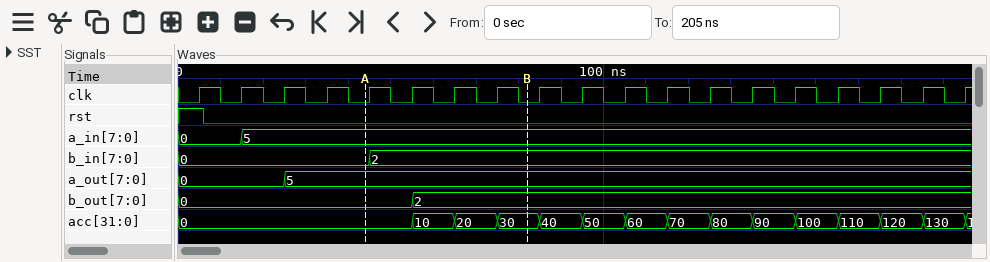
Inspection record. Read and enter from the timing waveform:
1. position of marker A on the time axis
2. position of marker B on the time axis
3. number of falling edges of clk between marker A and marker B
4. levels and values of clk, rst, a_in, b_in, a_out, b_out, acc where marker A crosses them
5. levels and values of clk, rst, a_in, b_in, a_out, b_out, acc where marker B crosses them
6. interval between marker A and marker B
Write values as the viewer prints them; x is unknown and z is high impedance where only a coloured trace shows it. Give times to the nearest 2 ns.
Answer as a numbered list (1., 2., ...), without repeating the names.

1. 44 ns
2. 82 ns
3. 4
4. clk=0, rst=0, a_in=5, b_in=0, a_out=5, b_out=0, acc=0
5. clk=0, rst=0, a_in=5, b_in=2, a_out=5, b_out=2, acc=30
6. 38 ns
